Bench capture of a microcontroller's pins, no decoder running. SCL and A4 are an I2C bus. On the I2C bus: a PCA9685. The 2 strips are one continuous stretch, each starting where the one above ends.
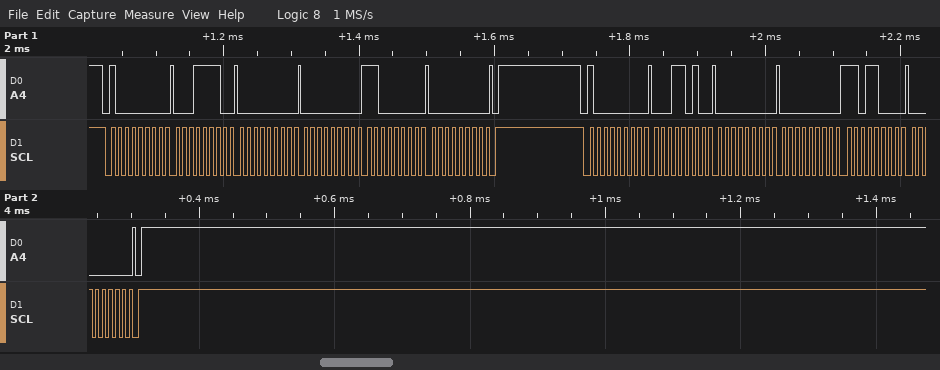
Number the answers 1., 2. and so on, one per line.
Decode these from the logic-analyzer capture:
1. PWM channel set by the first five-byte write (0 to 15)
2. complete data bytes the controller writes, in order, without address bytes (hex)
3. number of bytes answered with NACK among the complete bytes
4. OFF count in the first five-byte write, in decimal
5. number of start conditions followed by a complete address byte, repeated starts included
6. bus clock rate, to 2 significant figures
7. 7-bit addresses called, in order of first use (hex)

1. 6
2. 1E 00 00 C0 00 1A 00 00 D8 00
3. 0
4. 192
5. 2
6. 100 kHz
7. 0x40
